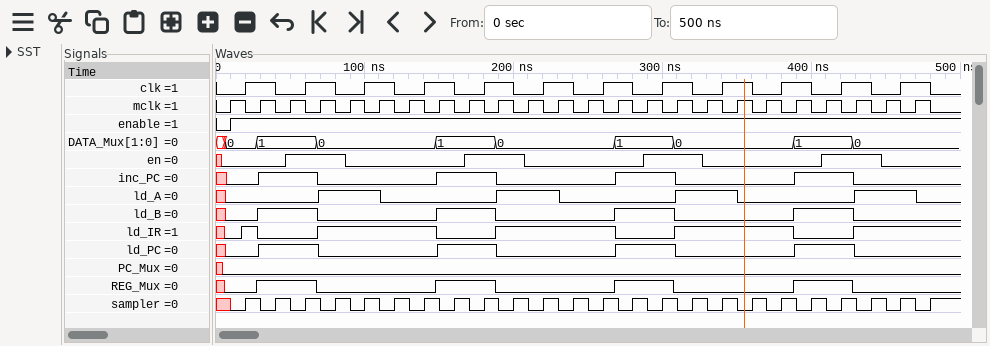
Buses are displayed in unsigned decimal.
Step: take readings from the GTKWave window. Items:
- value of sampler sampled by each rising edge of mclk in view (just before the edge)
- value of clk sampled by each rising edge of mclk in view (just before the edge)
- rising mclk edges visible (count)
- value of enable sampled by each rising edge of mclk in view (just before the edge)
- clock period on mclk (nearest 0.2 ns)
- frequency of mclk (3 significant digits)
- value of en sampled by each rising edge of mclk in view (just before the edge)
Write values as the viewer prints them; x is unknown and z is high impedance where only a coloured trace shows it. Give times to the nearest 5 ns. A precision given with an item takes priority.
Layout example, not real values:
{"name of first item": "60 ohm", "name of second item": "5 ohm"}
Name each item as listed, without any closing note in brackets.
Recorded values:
{"value of sampler sampled by each rising edge of mclk in view": "x 1 1 1 1 1 1 1 1 1 1 1 1 1 1 1 1 1 1 1 1 1 1 1", "value of clk sampled by each rising edge of mclk in view": "0 1 0 1 0 1 0 1 0 1 0 1 0 1 0 1 0 1 0 1 0 1 0 1", "rising mclk edges visible": "24", "value of enable sampled by each rising edge of mclk in view": "0 1 1 1 1 1 1 1 1 1 1 1 1 1 1 1 1 1 1 1 1 1 1 1", "clock period on mclk": "20 ns", "frequency of mclk": "50.0 MHz", "value of en sampled by each rising edge of mclk in view": "0 0 1 1 0 0 0 0 1 1 0 0 0 0 1 1 0 0 0 0 1 1 0 0"}
